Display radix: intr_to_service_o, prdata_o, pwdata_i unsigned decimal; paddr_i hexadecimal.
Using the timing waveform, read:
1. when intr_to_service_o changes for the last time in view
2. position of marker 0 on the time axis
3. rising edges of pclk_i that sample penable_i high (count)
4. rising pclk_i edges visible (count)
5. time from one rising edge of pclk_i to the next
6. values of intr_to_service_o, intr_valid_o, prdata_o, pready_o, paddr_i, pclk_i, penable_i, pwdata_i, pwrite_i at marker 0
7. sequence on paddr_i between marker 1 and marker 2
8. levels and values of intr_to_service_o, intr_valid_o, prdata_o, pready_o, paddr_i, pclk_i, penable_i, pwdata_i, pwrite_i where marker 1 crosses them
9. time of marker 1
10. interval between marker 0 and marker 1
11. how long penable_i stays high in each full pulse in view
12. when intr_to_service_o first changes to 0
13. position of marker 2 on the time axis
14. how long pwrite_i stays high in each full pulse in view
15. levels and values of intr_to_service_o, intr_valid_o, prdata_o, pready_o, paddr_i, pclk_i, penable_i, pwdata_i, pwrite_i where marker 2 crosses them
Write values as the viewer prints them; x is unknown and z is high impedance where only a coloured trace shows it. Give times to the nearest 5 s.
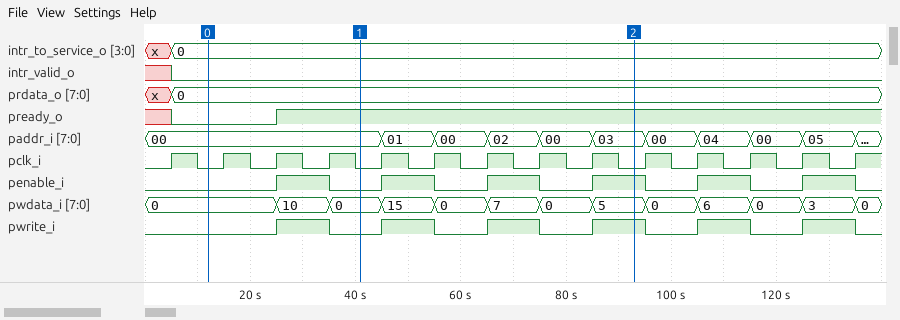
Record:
5 s
10 s
6
14
10 s
intr_to_service_o=0, intr_valid_o=0, prdata_o=0, pready_o=0, paddr_i=00, pclk_i=0, penable_i=0, pwdata_i=0, pwrite_i=0
00, 01, 00, 02, 00, 03
intr_to_service_o=0, intr_valid_o=0, prdata_o=0, pready_o=1, paddr_i=00, pclk_i=0, penable_i=0, pwdata_i=0, pwrite_i=0
40 s
30 s
10 s, 10 s, 10 s, 10 s, 10 s, 10 s
5 s
95 s
10 s, 10 s, 10 s, 10 s, 10 s, 10 s
intr_to_service_o=0, intr_valid_o=0, prdata_o=0, pready_o=1, paddr_i=03, pclk_i=0, penable_i=1, pwdata_i=5, pwrite_i=1
